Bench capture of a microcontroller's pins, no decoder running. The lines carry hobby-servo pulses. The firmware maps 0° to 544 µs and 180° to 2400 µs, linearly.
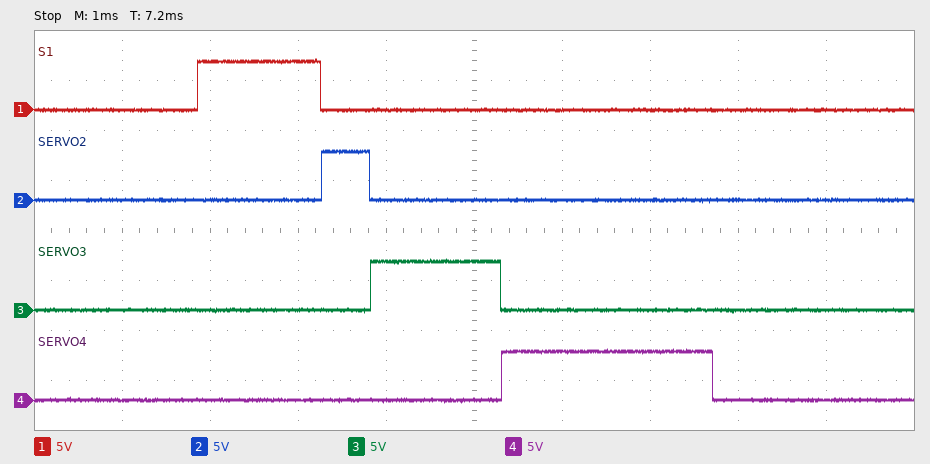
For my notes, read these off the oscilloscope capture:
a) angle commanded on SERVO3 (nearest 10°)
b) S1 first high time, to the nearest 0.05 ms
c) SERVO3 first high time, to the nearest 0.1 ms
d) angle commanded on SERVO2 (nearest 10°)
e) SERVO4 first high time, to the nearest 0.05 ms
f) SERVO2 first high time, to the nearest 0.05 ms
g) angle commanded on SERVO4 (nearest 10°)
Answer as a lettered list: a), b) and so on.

a) 90°
b) 1.40 ms
c) 1.5 ms
d) 0°
e) 2.40 ms
f) 0.55 ms
g) 180°
